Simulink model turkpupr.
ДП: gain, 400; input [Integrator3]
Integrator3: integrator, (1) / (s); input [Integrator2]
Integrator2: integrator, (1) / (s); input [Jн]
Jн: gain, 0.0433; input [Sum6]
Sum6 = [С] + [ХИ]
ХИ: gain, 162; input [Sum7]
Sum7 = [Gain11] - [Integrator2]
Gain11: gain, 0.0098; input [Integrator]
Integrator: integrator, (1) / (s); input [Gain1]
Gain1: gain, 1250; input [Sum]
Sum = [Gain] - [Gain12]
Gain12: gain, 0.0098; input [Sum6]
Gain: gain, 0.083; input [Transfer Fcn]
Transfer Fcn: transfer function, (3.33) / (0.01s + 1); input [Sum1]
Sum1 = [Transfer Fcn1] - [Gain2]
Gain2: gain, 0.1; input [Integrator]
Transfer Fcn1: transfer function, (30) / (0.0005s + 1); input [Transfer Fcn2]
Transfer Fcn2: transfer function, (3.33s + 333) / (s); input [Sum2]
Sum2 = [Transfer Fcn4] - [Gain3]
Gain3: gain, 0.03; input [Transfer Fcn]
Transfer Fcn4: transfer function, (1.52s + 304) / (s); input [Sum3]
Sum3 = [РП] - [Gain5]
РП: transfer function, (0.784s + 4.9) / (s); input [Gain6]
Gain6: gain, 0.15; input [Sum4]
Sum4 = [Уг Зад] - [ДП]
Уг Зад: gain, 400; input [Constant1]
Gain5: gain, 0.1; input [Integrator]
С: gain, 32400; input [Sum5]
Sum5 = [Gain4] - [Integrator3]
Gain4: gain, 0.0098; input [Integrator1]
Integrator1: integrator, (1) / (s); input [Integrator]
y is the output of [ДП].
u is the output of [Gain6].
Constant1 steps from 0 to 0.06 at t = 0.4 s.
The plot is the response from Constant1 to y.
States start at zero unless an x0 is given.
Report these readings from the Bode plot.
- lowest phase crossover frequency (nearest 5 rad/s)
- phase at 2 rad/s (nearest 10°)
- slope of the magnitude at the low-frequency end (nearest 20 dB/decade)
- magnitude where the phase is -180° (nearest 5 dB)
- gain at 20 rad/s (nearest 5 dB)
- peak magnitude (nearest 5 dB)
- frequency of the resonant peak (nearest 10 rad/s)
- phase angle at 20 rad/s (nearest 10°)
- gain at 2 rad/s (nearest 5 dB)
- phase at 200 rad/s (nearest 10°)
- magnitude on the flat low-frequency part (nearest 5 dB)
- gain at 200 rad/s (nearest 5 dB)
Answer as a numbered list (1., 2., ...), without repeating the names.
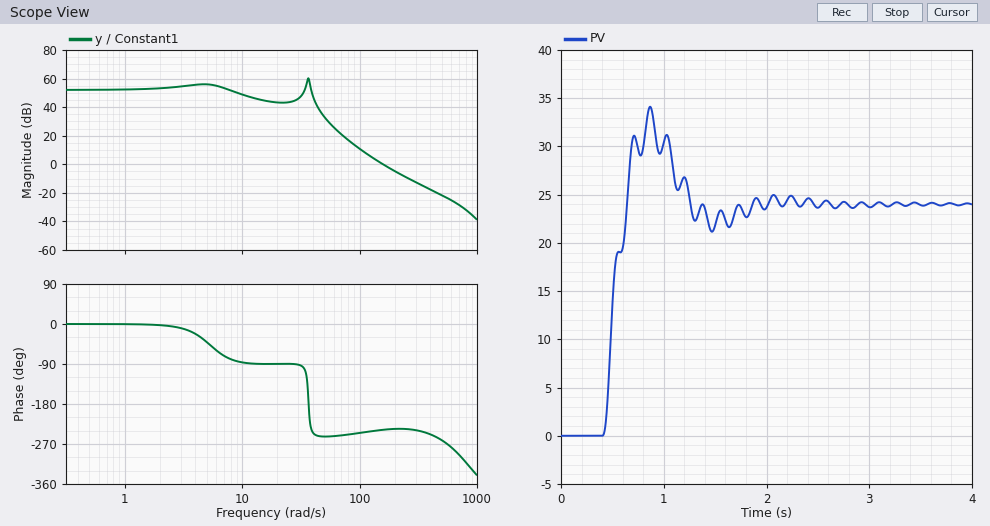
1. 35 rad/s
2. 0°
3. 0 dB/decade
4. 60 dB
5. 45 dB
6. 60 dB
7. 40 rad/s
8. -90°
9. 55 dB
10. -240°
11. 50 dB
12. -5 dB
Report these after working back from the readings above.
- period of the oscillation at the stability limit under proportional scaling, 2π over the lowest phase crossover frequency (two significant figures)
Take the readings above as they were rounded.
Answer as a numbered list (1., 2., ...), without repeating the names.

1. 0.18 s
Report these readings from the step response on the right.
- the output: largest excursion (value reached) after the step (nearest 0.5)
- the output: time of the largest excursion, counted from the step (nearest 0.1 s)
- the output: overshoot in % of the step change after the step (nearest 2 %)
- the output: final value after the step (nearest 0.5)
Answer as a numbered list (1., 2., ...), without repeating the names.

1. 34.0
2. 0.5 s
3. 42 %
4. 24.0
